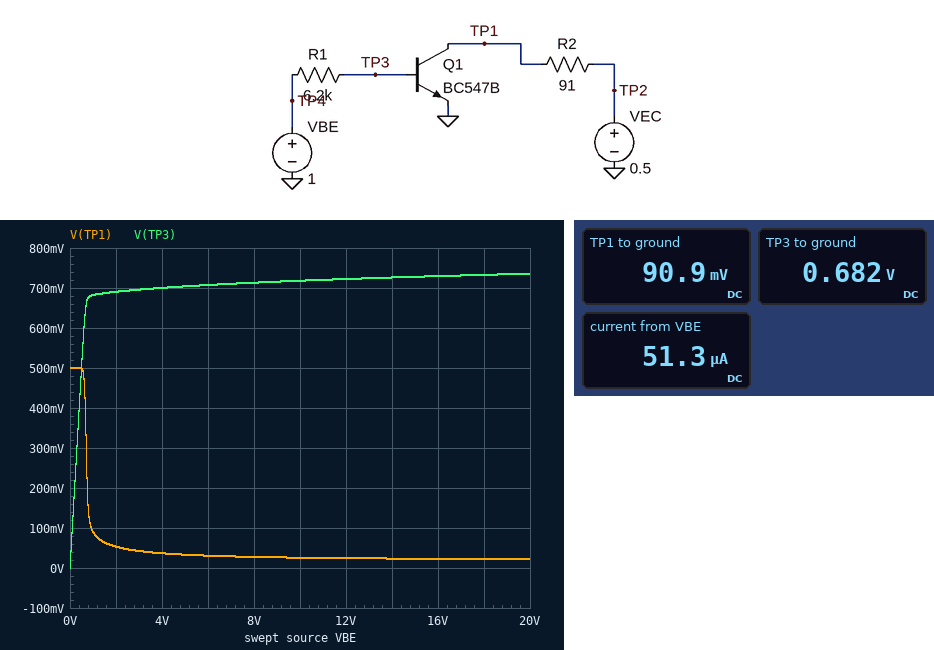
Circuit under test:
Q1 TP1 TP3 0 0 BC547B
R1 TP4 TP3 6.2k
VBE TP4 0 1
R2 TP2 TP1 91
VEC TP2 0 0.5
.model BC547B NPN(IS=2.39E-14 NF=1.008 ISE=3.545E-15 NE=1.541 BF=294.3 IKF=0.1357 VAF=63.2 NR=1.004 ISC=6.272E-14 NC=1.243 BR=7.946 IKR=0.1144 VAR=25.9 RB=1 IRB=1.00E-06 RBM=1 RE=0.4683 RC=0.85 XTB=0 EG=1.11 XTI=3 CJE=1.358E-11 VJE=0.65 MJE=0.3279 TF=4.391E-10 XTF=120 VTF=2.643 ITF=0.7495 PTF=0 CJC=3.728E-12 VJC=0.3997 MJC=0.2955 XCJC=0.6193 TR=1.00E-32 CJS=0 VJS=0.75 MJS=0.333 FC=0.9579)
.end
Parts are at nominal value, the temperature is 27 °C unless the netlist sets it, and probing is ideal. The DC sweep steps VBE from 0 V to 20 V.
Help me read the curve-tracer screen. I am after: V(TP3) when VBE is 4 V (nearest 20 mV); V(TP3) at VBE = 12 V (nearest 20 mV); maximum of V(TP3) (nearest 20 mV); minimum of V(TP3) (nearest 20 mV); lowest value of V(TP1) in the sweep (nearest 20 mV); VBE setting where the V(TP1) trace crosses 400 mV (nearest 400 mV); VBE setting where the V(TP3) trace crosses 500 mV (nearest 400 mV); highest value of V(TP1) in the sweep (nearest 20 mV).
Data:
700 mV
720 mV
740 mV
0 V
20 mV
800 mV
400 mV
500 mV
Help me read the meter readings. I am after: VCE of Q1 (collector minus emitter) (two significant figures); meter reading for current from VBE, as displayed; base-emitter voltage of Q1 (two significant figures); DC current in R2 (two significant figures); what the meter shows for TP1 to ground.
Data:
91 mV
51.3 µA
680 mV
4.5 mA
90.9 mV
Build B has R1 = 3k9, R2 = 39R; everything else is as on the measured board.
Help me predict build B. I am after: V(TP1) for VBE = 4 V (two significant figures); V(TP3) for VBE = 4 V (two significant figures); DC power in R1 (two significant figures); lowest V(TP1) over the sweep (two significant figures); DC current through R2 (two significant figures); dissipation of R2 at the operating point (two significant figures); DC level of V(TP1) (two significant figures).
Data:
53 mV
720 mV
22 µW
36 mV
9.8 mA
3.8 mW
120 mV
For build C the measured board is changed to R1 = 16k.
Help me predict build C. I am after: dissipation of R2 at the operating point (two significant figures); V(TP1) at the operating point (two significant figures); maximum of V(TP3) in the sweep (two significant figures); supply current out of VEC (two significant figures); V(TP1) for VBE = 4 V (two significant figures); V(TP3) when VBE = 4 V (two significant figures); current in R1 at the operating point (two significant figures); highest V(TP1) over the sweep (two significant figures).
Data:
1.5 mW
140 mV
710 mV
4.0 mA
54 mV
690 mV
20 µA
500 mV
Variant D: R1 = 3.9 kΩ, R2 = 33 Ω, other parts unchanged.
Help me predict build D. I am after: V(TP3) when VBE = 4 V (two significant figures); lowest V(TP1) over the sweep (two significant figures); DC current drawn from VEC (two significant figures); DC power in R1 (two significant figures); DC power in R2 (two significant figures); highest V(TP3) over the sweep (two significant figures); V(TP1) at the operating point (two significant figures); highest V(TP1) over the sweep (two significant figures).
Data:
730 mV
40 mV
11 mA
22 µW
4.2 mW
760 mV
130 mV
500 mV
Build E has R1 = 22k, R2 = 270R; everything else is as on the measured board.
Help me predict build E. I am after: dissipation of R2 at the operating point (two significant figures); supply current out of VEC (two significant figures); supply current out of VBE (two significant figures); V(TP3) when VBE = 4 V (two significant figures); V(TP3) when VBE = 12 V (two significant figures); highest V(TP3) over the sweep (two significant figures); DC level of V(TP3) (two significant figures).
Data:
620 µW
1.5 mA
16 µA
670 mV
690 mV
700 mV
650 mV
